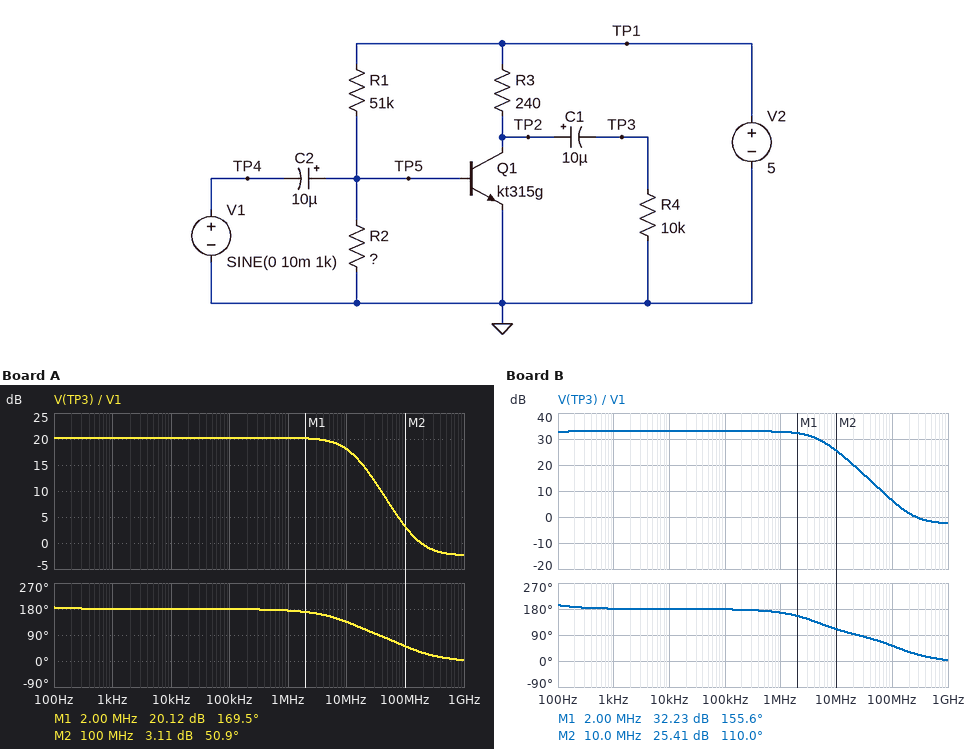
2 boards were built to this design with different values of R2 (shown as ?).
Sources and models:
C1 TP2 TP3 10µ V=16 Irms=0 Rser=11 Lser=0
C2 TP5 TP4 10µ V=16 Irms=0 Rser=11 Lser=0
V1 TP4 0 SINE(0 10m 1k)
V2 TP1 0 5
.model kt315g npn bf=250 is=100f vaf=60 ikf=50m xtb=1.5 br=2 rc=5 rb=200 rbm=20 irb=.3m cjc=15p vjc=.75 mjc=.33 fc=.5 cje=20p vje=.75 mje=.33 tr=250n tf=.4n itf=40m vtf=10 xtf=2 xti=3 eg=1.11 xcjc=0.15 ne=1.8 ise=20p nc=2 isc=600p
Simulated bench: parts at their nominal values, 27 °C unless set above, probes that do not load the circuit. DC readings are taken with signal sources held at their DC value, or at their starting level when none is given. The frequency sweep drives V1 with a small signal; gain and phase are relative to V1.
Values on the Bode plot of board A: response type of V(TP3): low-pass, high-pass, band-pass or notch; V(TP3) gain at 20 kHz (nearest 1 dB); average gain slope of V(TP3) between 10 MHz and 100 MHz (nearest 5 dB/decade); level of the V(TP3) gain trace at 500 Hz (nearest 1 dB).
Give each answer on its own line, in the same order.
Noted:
low-pass
20 dB
-15 dB/decade
20 dB
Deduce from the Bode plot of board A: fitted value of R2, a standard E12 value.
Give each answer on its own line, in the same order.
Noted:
8.2 kΩ
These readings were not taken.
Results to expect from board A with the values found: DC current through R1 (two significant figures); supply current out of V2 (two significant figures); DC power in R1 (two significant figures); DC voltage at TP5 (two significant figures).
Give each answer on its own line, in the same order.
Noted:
86 µA
1.3 mA
380 µW
600 mV
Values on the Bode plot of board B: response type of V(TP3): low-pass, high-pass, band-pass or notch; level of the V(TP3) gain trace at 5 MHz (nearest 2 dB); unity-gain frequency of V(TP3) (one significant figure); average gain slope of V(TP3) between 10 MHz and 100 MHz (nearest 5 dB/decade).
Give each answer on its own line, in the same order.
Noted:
low-pass
30 dB
300 MHz
-20 dB/decade
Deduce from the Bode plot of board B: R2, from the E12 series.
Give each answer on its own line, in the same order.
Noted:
22 kΩ
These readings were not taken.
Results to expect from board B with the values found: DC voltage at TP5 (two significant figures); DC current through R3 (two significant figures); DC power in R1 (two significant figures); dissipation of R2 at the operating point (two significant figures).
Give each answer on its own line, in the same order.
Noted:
660 mV
7.4 mA
370 µW
20 µW
